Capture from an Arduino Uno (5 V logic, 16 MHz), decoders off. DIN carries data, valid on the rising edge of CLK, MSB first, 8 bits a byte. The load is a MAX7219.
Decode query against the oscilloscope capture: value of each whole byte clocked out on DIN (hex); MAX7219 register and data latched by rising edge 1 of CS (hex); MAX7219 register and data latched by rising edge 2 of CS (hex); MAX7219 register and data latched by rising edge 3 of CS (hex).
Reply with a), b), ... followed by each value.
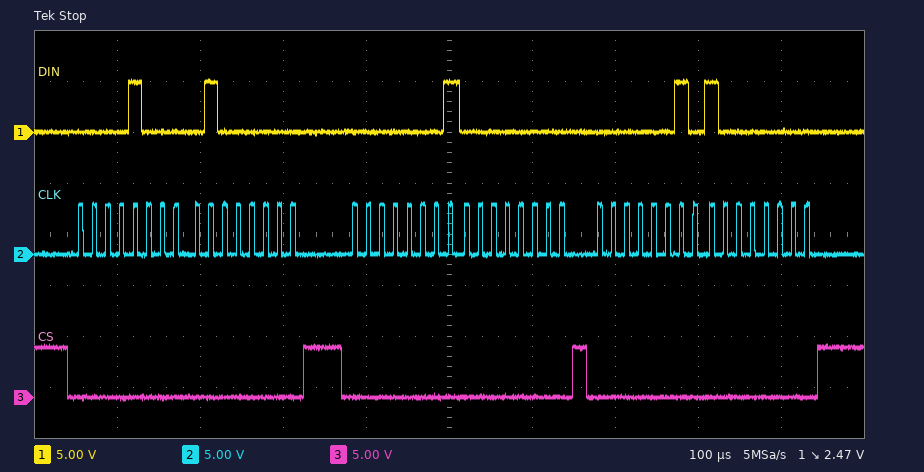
a) 08 40 01 00 02 80
b) register 0x8, data 0x40
c) register 0x1, data 0x00
d) register 0x2, data 0x80
